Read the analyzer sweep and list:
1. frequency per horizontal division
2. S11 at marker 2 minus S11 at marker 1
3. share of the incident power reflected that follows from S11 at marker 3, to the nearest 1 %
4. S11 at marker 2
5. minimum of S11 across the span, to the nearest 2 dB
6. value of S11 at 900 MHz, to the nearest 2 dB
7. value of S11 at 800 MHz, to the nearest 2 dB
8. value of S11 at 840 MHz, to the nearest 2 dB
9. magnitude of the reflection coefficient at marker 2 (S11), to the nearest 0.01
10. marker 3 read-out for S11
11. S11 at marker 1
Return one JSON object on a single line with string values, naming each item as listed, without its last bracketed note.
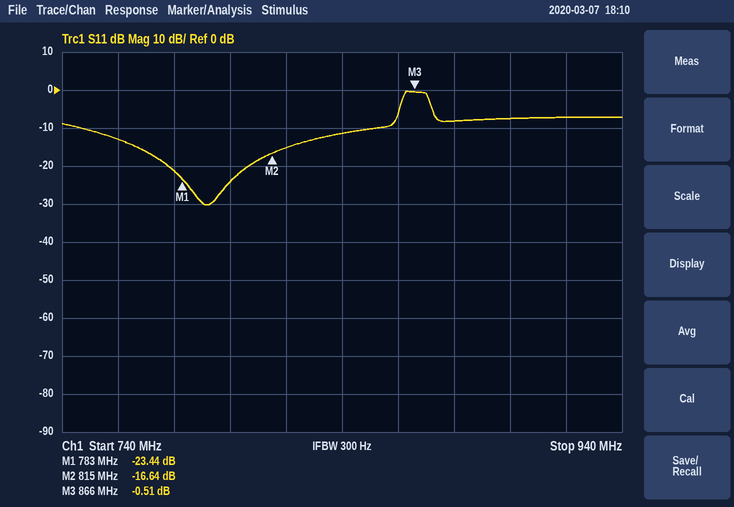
{"frequency per horizontal division": "20 MHz", "S11 at marker 2 minus S11 at marker 1": "6.80 dB", "share of the incident power reflected that follows from S11 at marker 3, to the nearest 1 %": "89 %", "S11 at marker 2": "-16.64 dB", "minimum of S11 across the span, to the nearest 2 dB": "-30 dB", "value of S11 at 900 MHz, to the nearest 2 dB": "-8 dB", "value of S11 at 800 MHz, to the nearest 2 dB": "-24 dB", "value of S11 at 840 MHz, to the nearest 2 dB": "-12 dB", "magnitude of the reflection coefficient at marker 2 (S11), to the nearest 0.01": "0.15", "marker 3 read-out for S11": "-0.51 dB", "S11 at marker 1": "-23.44 dB"}
